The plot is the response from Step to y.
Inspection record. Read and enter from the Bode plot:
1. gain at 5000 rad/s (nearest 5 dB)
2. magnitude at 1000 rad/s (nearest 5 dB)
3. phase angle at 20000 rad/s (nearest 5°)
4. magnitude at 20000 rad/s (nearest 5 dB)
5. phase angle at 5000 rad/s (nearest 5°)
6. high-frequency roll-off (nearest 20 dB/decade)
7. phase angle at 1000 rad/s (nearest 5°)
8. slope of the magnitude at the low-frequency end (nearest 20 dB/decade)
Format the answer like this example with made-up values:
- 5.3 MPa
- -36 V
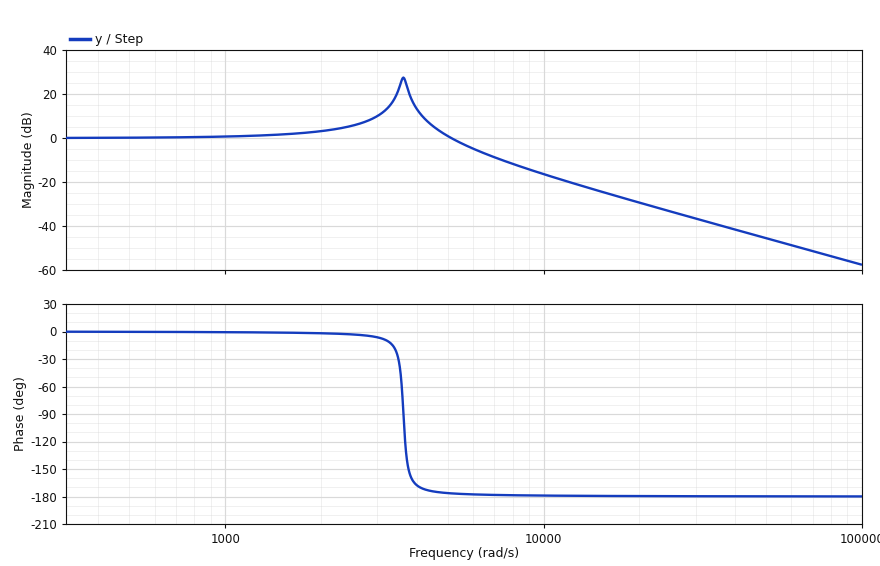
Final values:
- 0 dB
- 0 dB
- -180°
- -30 dB
- -175°
- -40 dB/decade
- 0°
- 0 dB/decade
